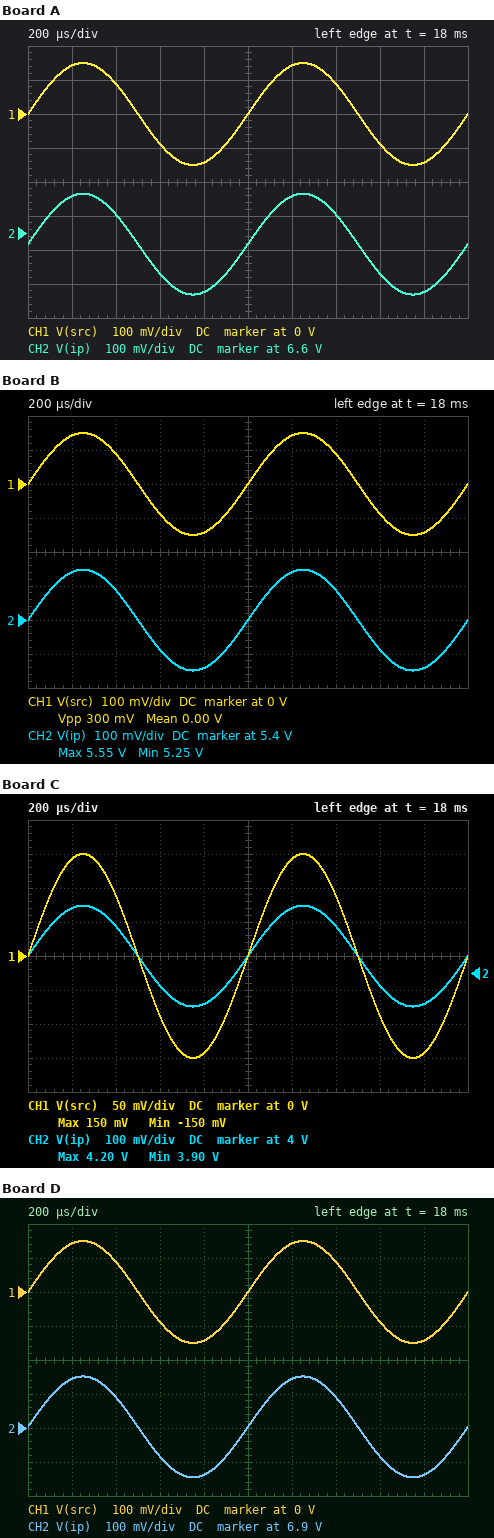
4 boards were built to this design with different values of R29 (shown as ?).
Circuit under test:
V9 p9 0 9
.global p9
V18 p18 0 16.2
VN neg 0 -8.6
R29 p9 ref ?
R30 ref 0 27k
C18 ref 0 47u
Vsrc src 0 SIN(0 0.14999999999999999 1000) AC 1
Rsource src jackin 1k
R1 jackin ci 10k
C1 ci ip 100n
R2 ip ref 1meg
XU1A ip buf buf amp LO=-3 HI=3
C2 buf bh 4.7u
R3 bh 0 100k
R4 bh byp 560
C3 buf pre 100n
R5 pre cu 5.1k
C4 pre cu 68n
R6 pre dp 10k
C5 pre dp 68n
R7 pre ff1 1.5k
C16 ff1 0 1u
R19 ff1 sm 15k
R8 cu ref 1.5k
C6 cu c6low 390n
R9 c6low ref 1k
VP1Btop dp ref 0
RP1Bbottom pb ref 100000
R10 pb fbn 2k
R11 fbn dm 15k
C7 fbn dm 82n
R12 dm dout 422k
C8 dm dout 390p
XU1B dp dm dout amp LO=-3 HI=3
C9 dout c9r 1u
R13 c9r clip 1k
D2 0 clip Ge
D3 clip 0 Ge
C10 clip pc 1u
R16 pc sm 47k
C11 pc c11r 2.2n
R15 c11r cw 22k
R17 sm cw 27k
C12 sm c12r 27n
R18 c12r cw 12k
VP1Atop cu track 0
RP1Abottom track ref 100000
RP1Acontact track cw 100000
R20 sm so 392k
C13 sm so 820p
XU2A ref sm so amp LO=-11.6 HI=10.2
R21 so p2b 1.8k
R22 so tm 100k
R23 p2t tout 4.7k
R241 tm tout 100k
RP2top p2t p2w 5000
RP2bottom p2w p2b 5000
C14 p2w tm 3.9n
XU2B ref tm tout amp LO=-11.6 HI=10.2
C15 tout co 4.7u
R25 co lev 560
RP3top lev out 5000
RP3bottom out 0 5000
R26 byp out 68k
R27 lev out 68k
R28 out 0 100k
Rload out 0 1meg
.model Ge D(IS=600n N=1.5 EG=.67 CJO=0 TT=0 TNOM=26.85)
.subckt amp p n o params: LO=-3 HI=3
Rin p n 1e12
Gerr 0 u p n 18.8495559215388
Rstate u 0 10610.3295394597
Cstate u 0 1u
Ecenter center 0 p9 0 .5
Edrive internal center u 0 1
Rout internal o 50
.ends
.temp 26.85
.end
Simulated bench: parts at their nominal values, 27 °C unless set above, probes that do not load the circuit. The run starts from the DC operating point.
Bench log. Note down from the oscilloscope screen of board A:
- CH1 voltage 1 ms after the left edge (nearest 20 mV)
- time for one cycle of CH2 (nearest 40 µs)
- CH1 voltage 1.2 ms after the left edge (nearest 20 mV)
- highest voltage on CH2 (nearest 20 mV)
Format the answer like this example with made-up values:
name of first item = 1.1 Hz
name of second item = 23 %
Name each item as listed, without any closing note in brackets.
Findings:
CH1 voltage 1 ms after the left edge = 0 V
time for one cycle of CH2 = 1.00 ms
CH1 voltage 1.2 ms after the left edge = 140 mV
highest voltage on CH2 = 6.72 V
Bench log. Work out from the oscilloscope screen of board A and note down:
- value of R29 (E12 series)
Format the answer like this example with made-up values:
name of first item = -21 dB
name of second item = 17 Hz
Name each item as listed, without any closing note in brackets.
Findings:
value of R29 = 10 kΩ
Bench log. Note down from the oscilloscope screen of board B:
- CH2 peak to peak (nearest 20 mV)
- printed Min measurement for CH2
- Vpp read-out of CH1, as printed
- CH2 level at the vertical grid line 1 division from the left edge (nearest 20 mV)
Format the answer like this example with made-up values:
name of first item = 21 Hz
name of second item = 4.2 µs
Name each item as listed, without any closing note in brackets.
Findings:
CH2 peak to peak = 300 mV
printed Min measurement for CH2 = 5.25 V
Vpp read-out of CH1, as printed = 300 mV
CH2 level at the vertical grid line 1 division from the left edge = 5.54 V
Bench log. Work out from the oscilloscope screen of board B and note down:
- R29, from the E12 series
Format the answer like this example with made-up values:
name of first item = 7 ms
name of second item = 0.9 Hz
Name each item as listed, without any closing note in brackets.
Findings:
R29, from the E12 series = 18 kΩ
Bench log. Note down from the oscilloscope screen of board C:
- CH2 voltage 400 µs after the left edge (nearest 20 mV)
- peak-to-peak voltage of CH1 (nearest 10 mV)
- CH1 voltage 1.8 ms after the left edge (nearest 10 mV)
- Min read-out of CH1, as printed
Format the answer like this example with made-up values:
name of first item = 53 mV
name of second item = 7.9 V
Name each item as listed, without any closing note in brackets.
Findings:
CH2 voltage 400 µs after the left edge = 4.14 V
peak-to-peak voltage of CH1 = 300 mV
CH1 voltage 1.8 ms after the left edge = -140 mV
Min read-out of CH1, as printed = -150 mV
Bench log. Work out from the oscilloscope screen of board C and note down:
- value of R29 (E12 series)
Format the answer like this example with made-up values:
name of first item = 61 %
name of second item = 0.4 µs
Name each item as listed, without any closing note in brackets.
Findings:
value of R29 = 33 kΩ
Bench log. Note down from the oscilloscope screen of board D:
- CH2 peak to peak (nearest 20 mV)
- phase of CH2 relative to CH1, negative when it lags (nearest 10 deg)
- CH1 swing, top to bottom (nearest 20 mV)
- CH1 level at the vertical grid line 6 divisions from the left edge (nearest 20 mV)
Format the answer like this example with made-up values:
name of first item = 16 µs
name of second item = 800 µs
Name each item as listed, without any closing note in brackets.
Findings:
CH2 peak to peak = 300 mV
phase of CH2 relative to CH1, negative when it lags = 0 deg
CH1 swing, top to bottom = 300 mV
CH1 level at the vertical grid line 6 divisions from the left edge = 140 mV
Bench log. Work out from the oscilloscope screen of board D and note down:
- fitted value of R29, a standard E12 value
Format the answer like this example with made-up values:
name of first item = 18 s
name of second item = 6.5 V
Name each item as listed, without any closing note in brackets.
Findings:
fitted value of R29, a standard E12 value = 8.2 kΩ
